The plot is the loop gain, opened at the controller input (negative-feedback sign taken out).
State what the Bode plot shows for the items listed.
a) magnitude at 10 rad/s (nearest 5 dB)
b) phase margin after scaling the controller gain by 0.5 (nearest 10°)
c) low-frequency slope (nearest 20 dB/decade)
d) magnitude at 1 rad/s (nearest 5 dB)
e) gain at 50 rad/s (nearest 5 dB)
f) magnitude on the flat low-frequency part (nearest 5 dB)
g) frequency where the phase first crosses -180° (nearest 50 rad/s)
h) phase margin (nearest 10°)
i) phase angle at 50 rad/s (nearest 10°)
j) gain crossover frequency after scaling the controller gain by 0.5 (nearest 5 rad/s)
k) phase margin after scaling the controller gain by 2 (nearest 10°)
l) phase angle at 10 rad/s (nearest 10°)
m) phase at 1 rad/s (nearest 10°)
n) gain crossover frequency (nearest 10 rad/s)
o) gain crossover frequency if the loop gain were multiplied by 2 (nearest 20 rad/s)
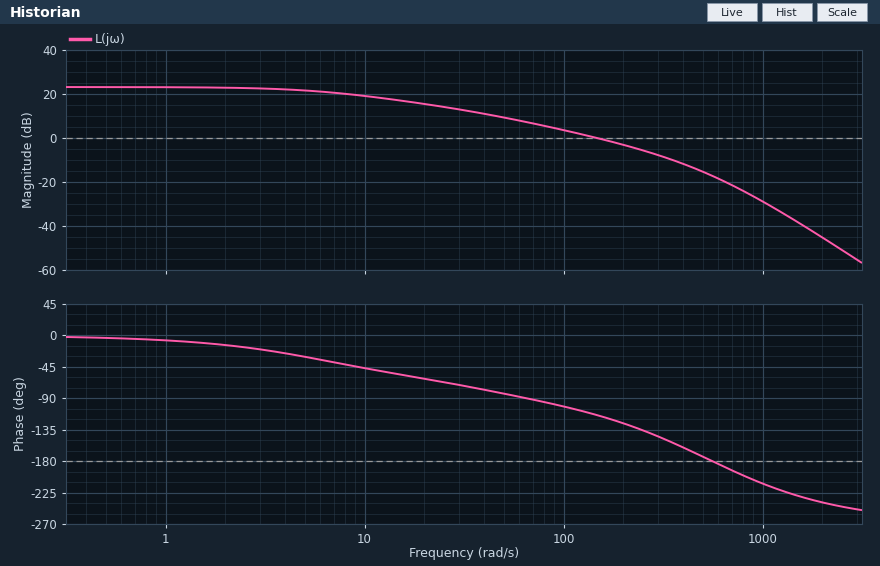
20 dB
90°
0 dB/decade
25 dB
10 dB
25 dB
550 rad/s
70°
-80°
75 rad/s
40°
-50°
-10°
150 rad/s
260 rad/s
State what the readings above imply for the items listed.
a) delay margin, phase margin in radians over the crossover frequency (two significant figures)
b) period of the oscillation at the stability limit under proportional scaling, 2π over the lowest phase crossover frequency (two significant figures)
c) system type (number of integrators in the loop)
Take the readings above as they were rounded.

0.0081 s
0.011 s
0
